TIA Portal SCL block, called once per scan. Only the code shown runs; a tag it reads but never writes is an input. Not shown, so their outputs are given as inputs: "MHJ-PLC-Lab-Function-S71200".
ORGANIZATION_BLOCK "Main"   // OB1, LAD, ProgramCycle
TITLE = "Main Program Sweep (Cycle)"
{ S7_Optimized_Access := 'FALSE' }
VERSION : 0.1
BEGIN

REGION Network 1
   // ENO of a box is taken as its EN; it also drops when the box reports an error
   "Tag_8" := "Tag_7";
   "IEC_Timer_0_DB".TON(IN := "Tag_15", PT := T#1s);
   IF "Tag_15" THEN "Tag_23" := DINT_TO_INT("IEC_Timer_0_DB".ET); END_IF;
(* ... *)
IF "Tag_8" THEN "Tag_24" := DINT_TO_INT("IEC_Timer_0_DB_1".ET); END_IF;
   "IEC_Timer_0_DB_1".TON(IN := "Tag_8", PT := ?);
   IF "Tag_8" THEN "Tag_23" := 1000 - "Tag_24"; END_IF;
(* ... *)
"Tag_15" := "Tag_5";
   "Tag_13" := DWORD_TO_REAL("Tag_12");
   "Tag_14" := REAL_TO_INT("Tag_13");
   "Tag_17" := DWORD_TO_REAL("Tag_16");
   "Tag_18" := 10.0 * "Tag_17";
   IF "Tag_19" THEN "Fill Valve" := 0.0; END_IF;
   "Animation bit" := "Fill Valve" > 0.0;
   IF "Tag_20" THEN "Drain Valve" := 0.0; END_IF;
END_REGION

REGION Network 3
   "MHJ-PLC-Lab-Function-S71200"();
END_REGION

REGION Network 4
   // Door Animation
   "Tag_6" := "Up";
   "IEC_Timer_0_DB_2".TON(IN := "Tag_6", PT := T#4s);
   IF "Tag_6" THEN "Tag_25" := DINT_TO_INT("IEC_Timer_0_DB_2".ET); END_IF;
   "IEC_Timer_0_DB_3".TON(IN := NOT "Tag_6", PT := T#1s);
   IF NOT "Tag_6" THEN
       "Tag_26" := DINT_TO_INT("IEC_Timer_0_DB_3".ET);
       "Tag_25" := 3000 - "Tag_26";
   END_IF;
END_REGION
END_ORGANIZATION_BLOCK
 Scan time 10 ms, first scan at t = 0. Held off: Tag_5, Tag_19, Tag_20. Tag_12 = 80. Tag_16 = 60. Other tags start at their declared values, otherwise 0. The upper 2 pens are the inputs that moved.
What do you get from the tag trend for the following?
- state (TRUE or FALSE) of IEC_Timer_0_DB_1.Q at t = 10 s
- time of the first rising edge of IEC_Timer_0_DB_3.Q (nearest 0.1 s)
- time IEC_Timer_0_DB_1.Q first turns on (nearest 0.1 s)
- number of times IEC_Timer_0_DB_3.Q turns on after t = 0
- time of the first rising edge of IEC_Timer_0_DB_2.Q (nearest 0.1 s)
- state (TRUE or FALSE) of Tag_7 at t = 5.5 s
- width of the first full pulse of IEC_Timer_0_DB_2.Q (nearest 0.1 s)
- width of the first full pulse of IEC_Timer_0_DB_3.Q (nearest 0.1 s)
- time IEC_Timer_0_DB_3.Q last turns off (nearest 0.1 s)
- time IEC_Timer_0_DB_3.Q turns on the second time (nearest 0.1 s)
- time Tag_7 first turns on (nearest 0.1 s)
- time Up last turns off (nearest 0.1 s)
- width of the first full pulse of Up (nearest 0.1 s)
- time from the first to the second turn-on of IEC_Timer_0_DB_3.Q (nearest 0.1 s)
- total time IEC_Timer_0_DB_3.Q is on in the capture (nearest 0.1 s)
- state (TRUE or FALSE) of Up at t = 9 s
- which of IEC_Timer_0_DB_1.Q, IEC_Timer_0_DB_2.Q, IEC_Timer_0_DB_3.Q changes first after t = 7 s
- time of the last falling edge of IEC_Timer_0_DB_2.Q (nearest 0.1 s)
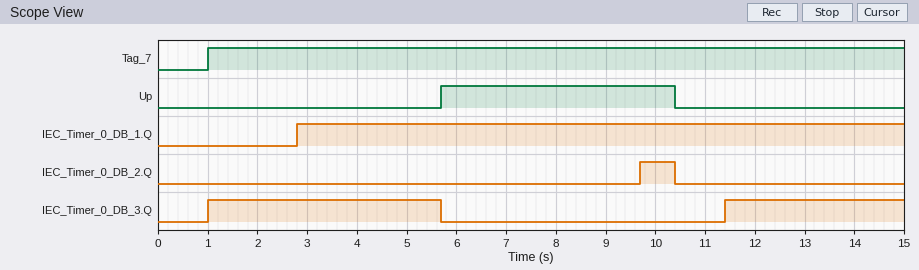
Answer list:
TRUE
1.0 s
2.8 s
2
9.7 s
TRUE
0.7 s
4.7 s
5.7 s
11.4 s
1.0 s
10.4 s
4.7 s
10.4 s
8.3 s
TRUE
IEC_Timer_0_DB_2.Q
10.4 s
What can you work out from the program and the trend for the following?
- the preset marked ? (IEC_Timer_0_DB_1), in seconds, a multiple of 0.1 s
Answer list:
1.8 s
